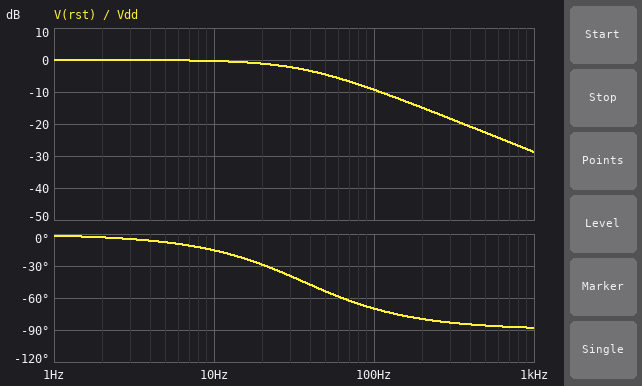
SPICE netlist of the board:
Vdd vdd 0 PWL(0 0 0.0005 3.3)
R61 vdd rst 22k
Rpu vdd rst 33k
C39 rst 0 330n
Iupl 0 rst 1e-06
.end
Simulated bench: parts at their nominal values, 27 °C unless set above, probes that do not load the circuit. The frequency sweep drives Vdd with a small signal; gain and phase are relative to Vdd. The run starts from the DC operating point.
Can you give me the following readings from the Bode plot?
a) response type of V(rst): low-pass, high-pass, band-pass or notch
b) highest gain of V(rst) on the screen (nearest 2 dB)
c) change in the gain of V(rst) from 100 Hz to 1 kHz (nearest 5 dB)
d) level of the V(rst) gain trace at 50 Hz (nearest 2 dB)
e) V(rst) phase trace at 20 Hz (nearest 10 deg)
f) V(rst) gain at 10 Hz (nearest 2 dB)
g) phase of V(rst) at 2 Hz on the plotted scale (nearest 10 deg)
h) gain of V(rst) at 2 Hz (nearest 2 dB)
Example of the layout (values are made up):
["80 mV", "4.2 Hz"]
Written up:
["low-pass", "0 dB", "-20 dB", "-4 dB", "-30 deg", "0 dB", "0 deg", "0 dB"]
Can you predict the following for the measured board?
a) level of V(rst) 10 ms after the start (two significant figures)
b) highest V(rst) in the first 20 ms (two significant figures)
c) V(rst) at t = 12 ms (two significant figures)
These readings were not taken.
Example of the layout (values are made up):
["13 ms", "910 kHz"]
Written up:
["3.0 V", "3.3 V", "3.1 V"]
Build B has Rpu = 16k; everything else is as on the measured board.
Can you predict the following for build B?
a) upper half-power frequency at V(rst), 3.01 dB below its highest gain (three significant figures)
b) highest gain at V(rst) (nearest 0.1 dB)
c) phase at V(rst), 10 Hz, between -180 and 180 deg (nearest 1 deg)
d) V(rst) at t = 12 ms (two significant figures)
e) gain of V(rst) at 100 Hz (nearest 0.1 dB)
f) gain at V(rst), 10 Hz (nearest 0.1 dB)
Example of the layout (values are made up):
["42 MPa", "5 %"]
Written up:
["52.1 Hz", "0 dB", "-11 deg", "3.2 V", "-6.7 dB", "-0.2 dB"]
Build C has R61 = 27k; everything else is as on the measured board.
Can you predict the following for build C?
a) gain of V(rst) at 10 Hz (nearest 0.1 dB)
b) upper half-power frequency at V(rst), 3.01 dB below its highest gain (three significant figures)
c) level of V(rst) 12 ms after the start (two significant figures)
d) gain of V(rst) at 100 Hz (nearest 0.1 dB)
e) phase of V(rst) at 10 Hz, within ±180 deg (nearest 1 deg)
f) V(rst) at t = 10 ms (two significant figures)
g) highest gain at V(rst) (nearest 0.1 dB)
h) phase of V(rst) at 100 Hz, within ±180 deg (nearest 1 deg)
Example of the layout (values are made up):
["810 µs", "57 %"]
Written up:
["-0.4 dB", "32.5 Hz", "3.0 V", "-10.2 dB", "-17 deg", "2.9 V", "0 dB", "-72 deg"]
